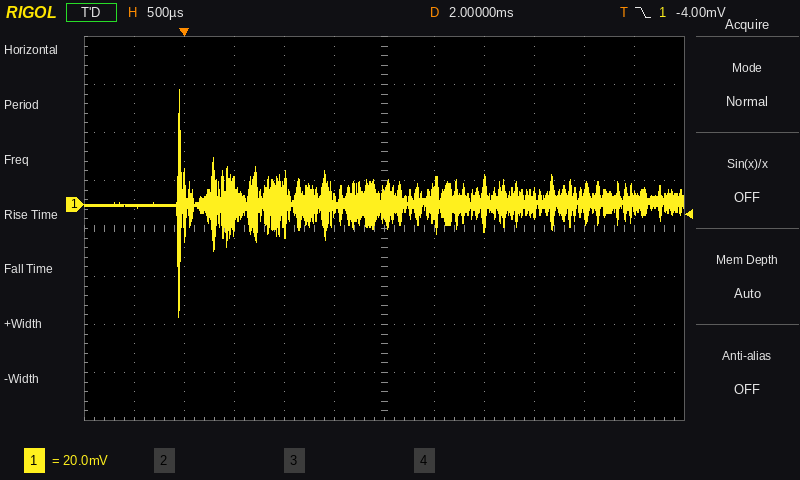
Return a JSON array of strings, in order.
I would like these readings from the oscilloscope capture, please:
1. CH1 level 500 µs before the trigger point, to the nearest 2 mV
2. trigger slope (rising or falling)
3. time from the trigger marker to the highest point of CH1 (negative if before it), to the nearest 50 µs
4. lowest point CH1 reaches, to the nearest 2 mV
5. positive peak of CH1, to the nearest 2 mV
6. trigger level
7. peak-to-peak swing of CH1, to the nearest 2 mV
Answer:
["0 mV", "falling", "-50 µs", "-48 mV", "48 mV", "-4.00 mV", "96 mV"]
